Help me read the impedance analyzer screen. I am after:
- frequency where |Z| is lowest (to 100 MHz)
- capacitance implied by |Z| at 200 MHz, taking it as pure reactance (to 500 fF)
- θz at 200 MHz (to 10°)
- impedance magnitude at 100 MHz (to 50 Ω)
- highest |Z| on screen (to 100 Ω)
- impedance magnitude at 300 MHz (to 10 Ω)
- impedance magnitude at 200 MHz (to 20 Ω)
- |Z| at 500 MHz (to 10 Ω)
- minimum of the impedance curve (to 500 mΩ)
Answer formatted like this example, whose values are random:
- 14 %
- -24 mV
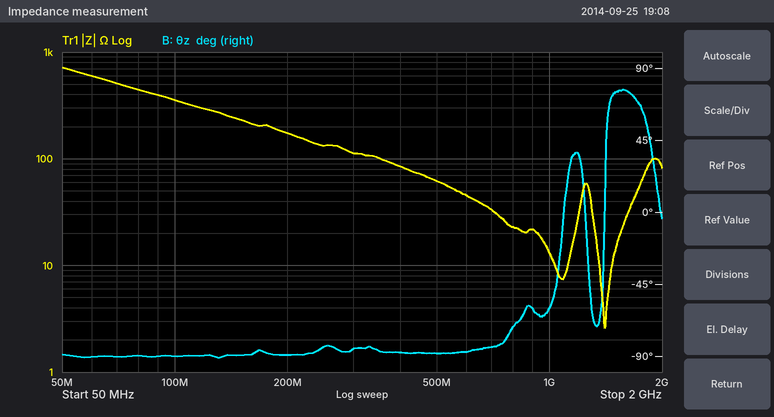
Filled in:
- 1.4 GHz
- 4.5 pF
- -90°
- 350 Ω
- 700 Ω
- 110 Ω
- 180 Ω
- 60 Ω
- 2.5 Ω
